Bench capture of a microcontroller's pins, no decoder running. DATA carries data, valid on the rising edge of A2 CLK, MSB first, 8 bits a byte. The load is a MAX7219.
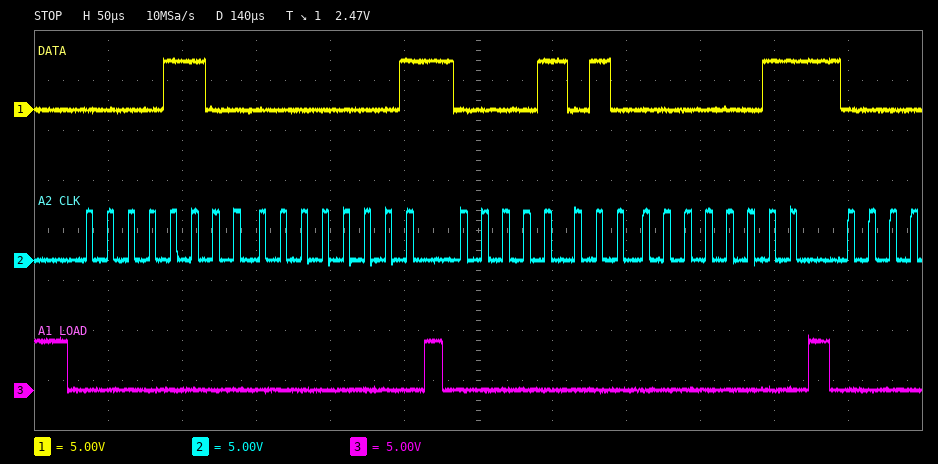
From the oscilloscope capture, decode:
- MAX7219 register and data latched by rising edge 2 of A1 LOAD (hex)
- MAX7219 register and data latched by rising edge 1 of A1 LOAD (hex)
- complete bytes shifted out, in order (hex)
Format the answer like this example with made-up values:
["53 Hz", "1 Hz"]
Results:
["register 0xA, data 0x03", "register 0xC, data 0x01", "0C 01 0A 03"]
